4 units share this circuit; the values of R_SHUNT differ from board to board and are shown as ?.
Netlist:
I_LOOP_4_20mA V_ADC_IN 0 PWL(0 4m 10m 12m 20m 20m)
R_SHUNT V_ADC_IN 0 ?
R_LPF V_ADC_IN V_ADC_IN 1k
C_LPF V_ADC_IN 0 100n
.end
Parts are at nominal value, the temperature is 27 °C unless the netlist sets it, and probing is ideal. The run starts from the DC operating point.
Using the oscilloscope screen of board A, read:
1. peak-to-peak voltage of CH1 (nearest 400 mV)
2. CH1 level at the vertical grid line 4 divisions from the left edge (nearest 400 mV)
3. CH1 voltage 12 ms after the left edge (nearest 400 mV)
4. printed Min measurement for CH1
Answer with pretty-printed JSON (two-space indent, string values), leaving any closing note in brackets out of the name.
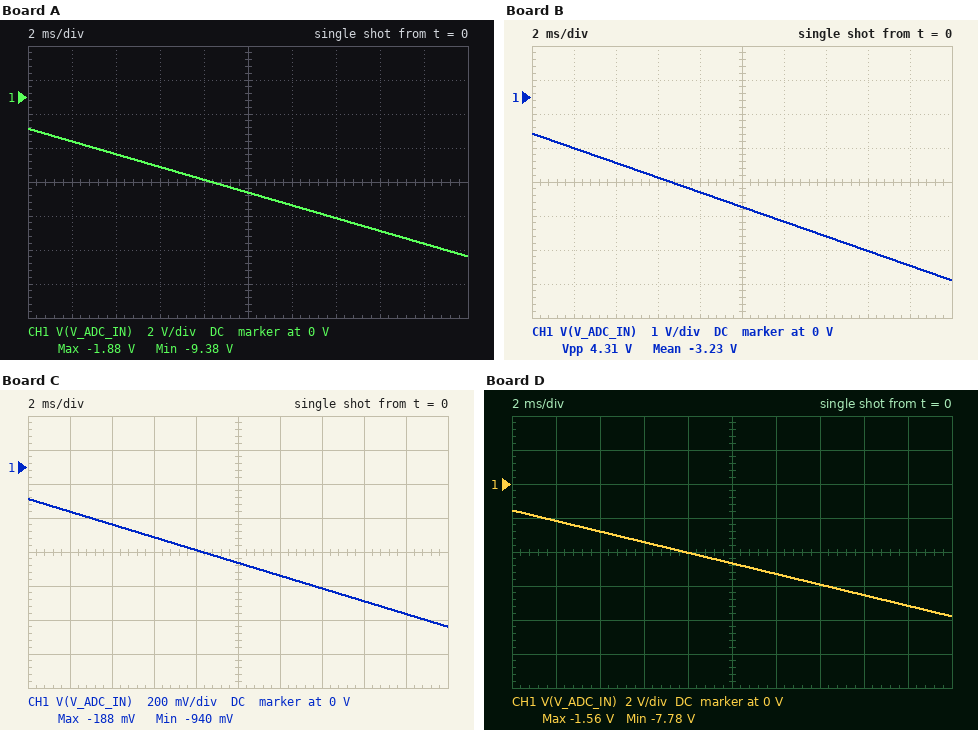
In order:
{
  "peak-to-peak voltage of CH1": "7.6 V",
  "CH1 level at the vertical grid line 4 divisions from the left edge": "-4.8 V",
  "CH1 voltage 12 ms after the left edge": "-6.4 V",
  "printed Min measurement for CH1": "-9.38 V"
}
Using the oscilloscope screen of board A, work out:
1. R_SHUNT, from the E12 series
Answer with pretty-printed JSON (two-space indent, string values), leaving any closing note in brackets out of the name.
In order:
{
  "R_SHUNT, from the E12 series": "470 Ω"
}
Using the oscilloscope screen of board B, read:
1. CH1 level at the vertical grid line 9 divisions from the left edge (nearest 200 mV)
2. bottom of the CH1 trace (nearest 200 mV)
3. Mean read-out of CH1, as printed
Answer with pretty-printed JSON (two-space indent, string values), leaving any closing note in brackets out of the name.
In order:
{
  "CH1 level at the vertical grid line 9 divisions from the left edge": "-5.0 V",
  "bottom of the CH1 trace": "-5.4 V",
  "Mean read-out of CH1, as printed": "-3.23 V"
}
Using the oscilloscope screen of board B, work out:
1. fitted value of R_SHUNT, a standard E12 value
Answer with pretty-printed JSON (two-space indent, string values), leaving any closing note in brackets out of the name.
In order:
{
  "fitted value of R_SHUNT, a standard E12 value": "270 Ω"
}
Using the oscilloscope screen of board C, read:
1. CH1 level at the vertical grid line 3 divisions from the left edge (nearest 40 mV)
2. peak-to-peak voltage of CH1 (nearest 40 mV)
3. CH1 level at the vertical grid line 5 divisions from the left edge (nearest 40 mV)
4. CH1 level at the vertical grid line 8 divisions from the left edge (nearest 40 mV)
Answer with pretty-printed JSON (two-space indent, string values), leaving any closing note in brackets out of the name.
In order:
{
  "CH1 level at the vertical grid line 3 divisions from the left edge": "-400 mV",
  "peak-to-peak voltage of CH1": "760 mV",
  "CH1 level at the vertical grid line 5 divisions from the left edge": "-560 mV",
  "CH1 level at the vertical grid line 8 divisions from the left edge": "-800 mV"
}
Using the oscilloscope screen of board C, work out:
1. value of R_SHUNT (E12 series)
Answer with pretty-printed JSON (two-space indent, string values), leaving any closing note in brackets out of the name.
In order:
{
  "value of R_SHUNT": "47 Ω"
}
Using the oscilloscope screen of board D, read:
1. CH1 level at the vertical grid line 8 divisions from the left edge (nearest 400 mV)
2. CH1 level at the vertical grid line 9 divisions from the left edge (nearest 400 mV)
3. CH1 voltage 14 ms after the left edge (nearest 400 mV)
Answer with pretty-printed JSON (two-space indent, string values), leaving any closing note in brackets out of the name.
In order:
{
  "CH1 level at the vertical grid line 8 divisions from the left edge": "-6.4 V",
  "CH1 level at the vertical grid line 9 divisions from the left edge": "-7.2 V",
  "CH1 voltage 14 ms after the left edge": "-6.0 V"
}
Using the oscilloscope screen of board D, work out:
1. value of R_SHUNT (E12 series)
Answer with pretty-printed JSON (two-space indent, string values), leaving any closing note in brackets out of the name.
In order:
{
  "value of R_SHUNT": "390 Ω"
}
